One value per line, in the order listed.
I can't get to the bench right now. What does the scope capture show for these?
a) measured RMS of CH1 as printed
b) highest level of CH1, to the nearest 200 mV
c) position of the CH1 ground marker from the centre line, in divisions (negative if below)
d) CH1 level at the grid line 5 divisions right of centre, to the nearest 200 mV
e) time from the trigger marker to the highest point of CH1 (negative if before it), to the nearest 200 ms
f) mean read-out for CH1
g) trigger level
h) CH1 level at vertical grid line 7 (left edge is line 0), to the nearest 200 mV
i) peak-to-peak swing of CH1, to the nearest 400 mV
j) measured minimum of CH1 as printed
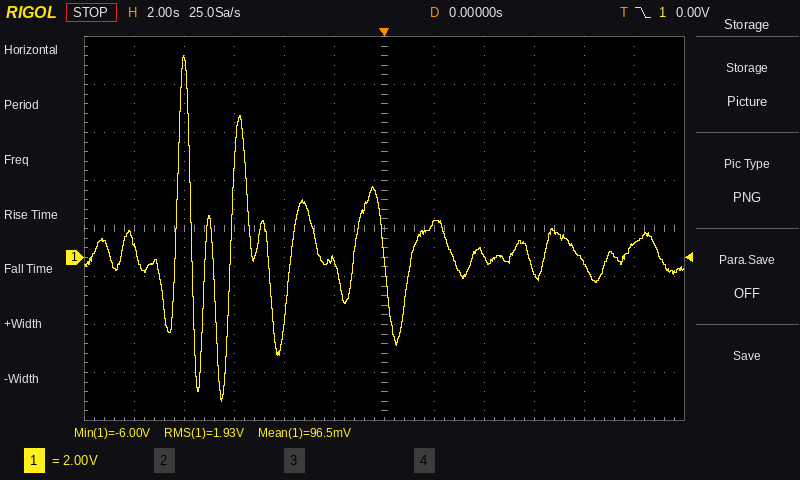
1.93 V
8.4 V
-0.6 div
600 mV
-8.0 s
96.5 mV
0.00 V
1.4 V
14.4 V
-6.00 V
